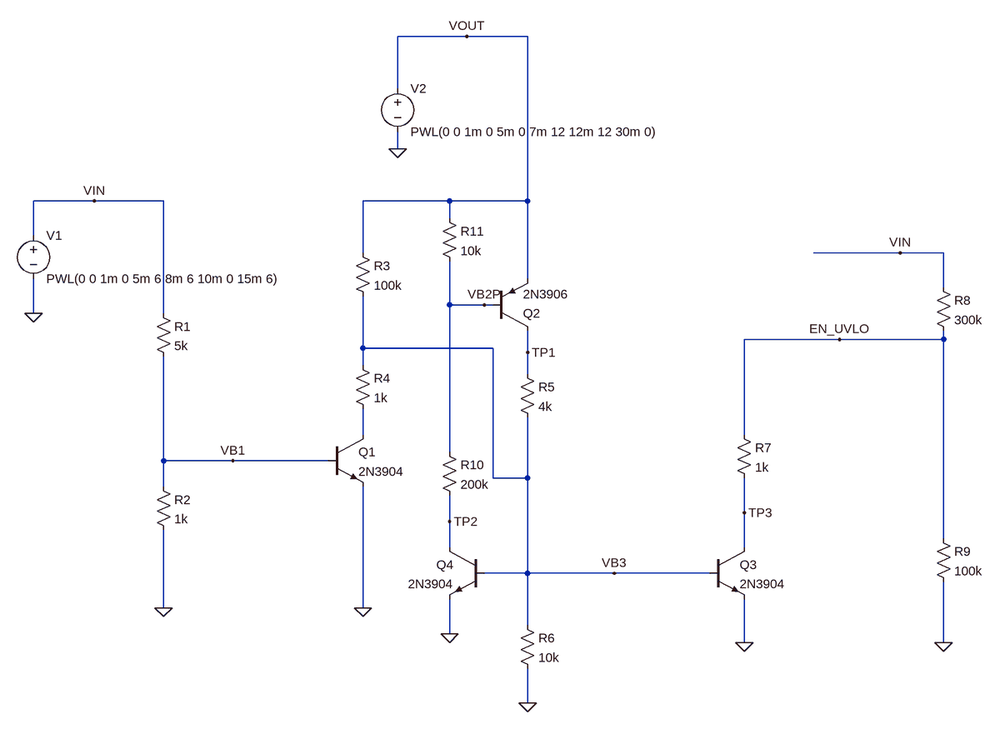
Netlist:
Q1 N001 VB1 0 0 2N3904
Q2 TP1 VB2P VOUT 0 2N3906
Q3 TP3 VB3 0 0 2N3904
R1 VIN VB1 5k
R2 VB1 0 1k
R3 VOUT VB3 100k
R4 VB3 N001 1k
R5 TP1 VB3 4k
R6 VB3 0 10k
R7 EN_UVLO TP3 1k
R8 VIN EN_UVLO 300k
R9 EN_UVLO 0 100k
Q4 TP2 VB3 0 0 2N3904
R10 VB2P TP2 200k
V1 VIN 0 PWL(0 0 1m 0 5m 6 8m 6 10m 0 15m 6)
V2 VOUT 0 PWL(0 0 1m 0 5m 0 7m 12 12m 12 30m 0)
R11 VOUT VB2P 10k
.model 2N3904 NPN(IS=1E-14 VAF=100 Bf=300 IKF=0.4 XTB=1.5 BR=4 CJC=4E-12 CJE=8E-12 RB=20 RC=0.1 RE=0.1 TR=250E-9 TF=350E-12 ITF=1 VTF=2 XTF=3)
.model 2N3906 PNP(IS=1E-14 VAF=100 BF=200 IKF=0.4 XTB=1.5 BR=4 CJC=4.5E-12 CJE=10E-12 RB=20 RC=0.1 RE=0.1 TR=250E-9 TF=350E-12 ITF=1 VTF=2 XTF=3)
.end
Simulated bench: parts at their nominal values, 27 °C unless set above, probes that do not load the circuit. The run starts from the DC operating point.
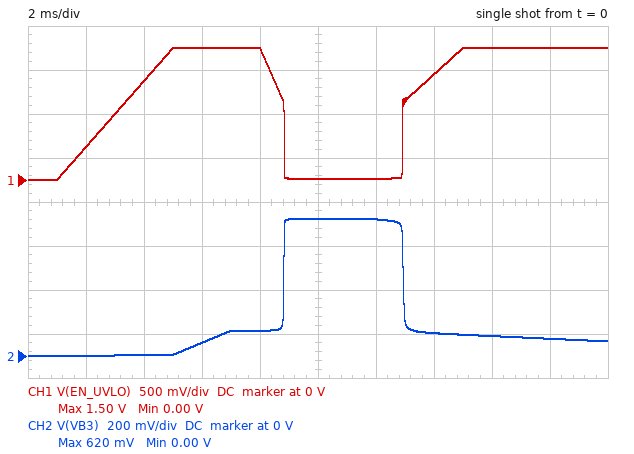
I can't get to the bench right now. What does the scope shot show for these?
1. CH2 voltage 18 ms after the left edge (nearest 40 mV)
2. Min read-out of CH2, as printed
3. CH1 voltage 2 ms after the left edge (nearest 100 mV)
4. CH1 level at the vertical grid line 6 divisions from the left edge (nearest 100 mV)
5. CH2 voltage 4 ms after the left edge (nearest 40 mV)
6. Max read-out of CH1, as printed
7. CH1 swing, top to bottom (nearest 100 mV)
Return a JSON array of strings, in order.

["80 mV", "0.00 V", "400 mV", "0 V", "0 V", "1.50 V", "1.5 V"]
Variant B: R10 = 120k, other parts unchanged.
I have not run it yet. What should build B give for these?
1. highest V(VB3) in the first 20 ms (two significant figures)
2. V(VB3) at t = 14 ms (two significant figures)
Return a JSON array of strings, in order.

["730 mV", "710 mV"]
